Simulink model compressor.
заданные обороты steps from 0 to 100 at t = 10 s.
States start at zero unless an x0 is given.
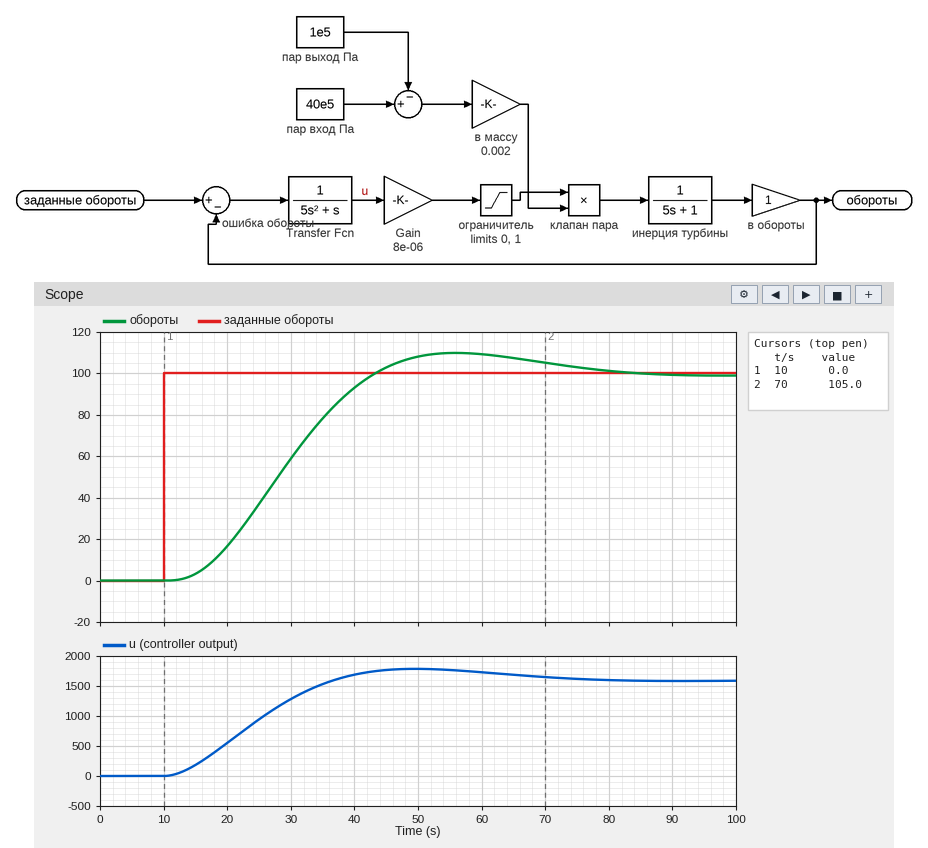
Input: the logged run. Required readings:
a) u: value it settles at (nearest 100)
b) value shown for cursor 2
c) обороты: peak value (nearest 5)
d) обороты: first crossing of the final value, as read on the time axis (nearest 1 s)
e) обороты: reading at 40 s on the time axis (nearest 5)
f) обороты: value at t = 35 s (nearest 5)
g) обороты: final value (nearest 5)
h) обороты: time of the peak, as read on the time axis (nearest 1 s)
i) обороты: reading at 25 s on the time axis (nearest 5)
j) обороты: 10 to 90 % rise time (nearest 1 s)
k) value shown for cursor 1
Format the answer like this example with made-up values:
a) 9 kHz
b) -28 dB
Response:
a) 1600
b) 105.0
c) 110
d) 43 s
e) 95
f) 80
g) 100
h) 56 s
i) 35
j) 21 s
k) 0.0
